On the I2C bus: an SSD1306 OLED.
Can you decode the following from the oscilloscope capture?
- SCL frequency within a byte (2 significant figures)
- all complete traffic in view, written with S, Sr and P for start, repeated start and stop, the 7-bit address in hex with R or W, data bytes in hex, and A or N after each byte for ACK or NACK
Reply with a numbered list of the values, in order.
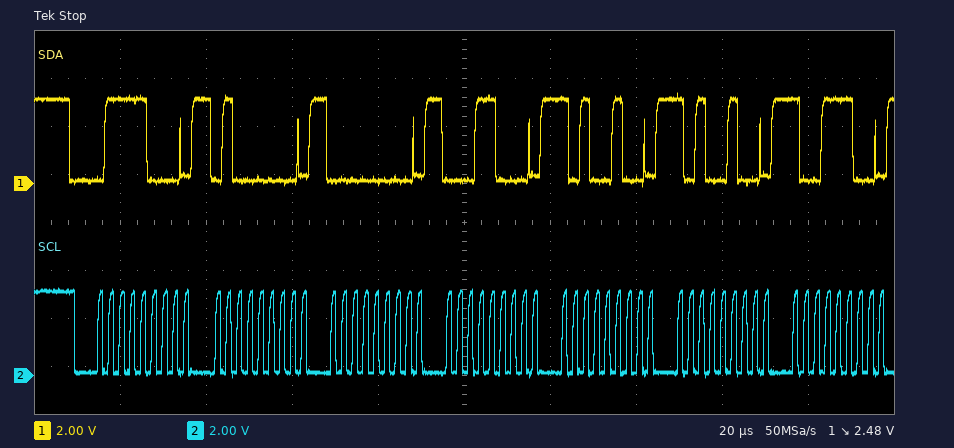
1. 400 kHz
2. S 3CW A 40 A 00 A 18 A A4 A A4 A 9C A
